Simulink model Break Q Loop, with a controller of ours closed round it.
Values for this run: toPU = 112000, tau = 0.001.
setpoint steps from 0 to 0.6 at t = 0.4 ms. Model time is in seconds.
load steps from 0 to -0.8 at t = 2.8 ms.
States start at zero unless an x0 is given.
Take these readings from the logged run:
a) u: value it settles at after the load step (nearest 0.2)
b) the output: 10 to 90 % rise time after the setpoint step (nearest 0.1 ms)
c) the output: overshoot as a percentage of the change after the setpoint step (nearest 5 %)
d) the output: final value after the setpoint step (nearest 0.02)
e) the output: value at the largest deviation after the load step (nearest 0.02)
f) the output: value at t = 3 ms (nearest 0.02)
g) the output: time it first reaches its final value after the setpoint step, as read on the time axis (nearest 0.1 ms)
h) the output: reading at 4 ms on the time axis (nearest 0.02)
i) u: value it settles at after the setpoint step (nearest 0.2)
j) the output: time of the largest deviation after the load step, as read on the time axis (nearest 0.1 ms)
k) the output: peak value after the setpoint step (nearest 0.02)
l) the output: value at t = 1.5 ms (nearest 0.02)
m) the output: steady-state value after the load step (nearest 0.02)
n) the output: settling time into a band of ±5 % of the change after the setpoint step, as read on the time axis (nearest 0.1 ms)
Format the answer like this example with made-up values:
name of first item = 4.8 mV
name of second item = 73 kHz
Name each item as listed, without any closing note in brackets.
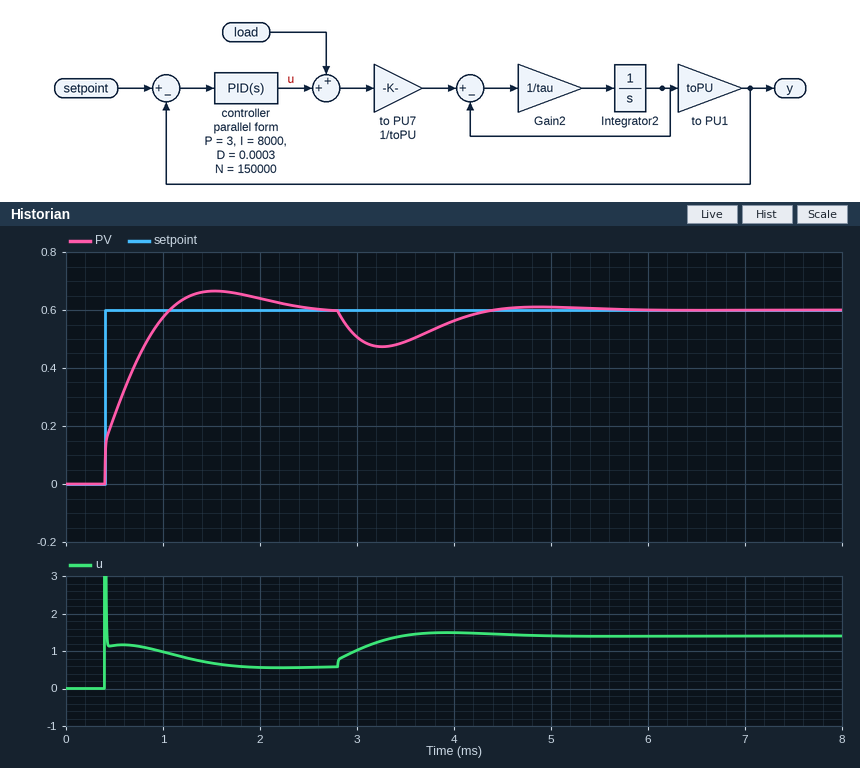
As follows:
u: value it settles at after the load step = 1.4
the output: 10 to 90 % rise time after the setpoint step = 0.5 ms
the output: overshoot as a percentage of the change after the setpoint step = 10 %
the output: final value after the setpoint step = 0.60
the output: value at the largest deviation after the load step = 0.48
the output: value at t = 3 ms = 0.50
the output: time it first reaches its final value after the setpoint step, as read on the time axis = 1.1 ms
the output: reading at 4 ms on the time axis = 0.56
u: value it settles at after the setpoint step = 0.6
the output: time of the largest deviation after the load step, as read on the time axis = 3.3 ms
the output: peak value after the setpoint step = 0.66
the output: value at t = 1.5 ms = 0.66
the output: steady-state value after the load step = 0.60
the output: settling time into a band of ±5 % of the change after the setpoint step, as read on the time axis = 2.1 ms
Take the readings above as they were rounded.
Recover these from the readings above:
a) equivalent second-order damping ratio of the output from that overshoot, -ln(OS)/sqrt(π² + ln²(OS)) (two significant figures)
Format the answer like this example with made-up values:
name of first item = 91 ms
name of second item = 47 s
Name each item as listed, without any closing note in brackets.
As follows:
equivalent second-order damping ratio of the output from that overshoot, -ln(OS)/sqrt(π² + ln²(OS)) = 0.59
